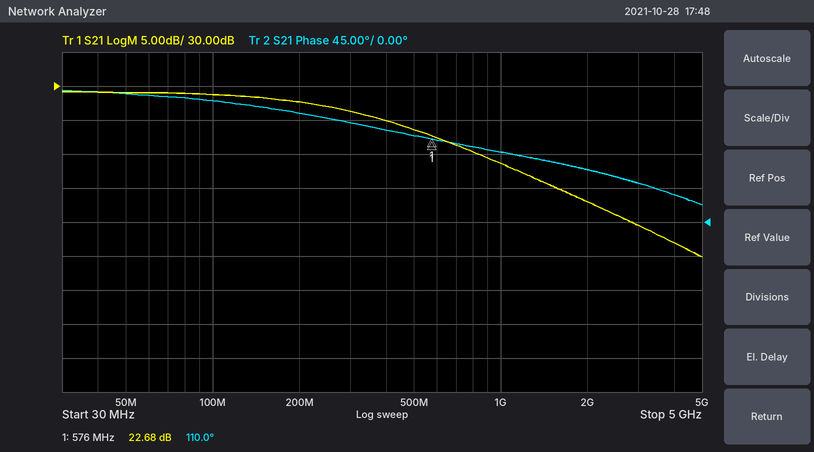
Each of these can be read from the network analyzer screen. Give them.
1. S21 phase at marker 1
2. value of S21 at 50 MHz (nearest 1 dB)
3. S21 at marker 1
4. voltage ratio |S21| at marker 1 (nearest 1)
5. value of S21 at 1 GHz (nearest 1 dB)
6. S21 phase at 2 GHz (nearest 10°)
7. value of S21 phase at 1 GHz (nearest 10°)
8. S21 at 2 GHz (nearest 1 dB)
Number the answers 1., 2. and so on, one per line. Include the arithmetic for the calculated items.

1. 110.0°
2. 29 dB
3. 22.68 dB
4. 10^(22.68/20) ≈ 14
5. 19 dB
6. 70°
7. 90°
8. 13 dB
